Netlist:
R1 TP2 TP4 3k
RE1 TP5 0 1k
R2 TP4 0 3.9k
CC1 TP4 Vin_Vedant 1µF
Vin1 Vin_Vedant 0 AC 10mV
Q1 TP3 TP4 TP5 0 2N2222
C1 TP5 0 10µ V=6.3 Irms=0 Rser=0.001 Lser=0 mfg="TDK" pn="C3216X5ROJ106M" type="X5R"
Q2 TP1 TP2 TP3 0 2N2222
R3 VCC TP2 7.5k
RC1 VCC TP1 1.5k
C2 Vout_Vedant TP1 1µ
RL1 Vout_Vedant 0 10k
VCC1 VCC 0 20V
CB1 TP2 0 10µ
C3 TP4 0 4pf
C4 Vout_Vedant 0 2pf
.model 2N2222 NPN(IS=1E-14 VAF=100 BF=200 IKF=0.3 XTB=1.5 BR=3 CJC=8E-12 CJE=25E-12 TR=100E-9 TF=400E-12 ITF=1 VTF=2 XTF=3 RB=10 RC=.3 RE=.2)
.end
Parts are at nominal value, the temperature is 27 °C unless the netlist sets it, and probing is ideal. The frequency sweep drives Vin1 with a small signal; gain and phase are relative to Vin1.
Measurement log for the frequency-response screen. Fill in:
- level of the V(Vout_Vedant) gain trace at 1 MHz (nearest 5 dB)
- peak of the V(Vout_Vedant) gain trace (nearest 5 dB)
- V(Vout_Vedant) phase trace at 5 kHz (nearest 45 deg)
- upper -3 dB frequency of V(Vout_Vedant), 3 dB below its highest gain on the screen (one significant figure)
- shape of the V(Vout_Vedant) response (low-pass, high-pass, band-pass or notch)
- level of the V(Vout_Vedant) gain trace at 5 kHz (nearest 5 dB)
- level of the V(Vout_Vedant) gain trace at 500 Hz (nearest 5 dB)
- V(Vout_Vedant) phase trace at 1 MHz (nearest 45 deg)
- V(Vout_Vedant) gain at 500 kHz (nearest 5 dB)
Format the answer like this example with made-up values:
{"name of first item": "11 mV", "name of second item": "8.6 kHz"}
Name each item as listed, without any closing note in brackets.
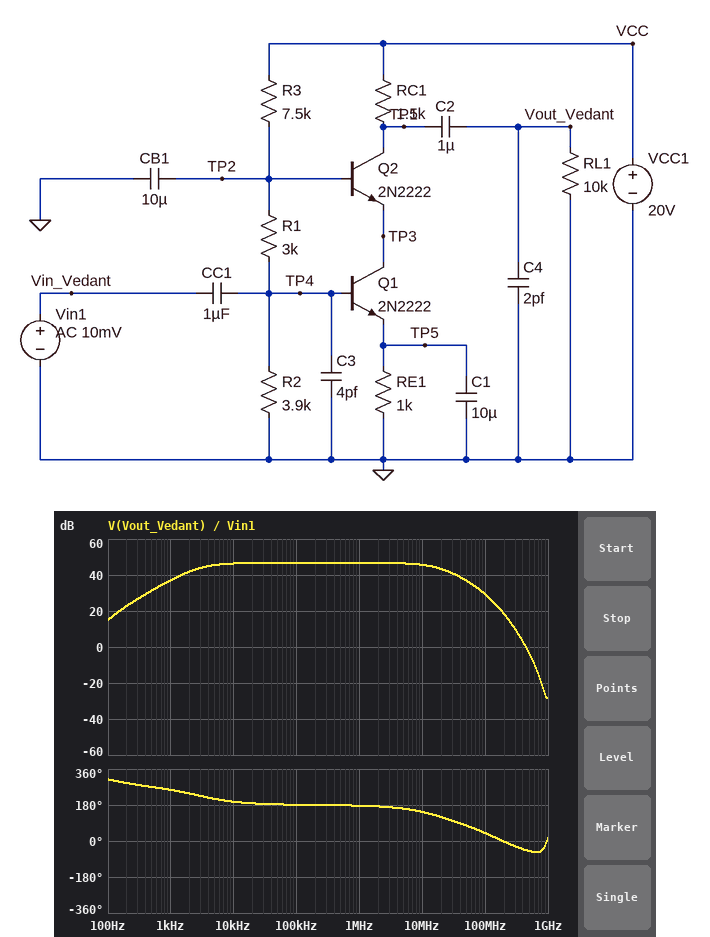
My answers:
{"level of the V(Vout_Vedant) gain trace at 1 MHz": "45 dB", "peak of the V(Vout_Vedant) gain trace": "45 dB", "V(Vout_Vedant) phase trace at 5 kHz": "225 deg", "upper -3 dB frequency of V(Vout_Vedant), 3 dB below its highest gain on the screen": "20 MHz", "shape of the V(Vout_Vedant) response": "band-pass", "level of the V(Vout_Vedant) gain trace at 5 kHz": "45 dB", "level of the V(Vout_Vedant) gain trace at 500 Hz": "30 dB", "V(Vout_Vedant) phase trace at 1 MHz": "180 deg", "V(Vout_Vedant) gain at 500 kHz": "45 dB"}
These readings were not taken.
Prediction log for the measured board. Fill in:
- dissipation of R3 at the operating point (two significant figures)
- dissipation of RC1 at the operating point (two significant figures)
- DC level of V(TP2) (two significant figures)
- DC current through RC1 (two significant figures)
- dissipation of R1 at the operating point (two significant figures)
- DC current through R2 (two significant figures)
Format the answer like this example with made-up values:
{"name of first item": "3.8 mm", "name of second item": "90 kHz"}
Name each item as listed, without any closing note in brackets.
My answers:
{"dissipation of R3 at the operating point": "15 mW", "dissipation of RC1 at the operating point": "31 mW", "DC level of V(TP2)": "9.5 V", "DC current through RC1": "4.6 mA", "dissipation of R1 at the operating point": "5.7 mW", "DC current through R2": "1.4 mA"}
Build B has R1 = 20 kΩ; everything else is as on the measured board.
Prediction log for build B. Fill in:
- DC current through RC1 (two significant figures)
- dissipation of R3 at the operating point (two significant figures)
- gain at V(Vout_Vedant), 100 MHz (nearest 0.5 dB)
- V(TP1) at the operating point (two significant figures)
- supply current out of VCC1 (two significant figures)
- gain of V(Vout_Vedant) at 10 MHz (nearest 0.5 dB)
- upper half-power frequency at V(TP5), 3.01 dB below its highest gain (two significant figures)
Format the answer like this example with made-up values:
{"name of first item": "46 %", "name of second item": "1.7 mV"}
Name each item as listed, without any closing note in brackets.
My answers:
{"DC current through RC1": "1.8 mA", "dissipation of R3 at the operating point": "3.1 mW", "gain at V(Vout_Vedant), 100 MHz": "21.0 dB", "V(TP1) at the operating point": "17 V", "supply current out of VCC1": "2.4 mA", "gain of V(Vout_Vedant) at 10 MHz": "37.5 dB", "upper half-power frequency at V(TP5), 3.01 dB below its highest gain": "1.2 kHz"}
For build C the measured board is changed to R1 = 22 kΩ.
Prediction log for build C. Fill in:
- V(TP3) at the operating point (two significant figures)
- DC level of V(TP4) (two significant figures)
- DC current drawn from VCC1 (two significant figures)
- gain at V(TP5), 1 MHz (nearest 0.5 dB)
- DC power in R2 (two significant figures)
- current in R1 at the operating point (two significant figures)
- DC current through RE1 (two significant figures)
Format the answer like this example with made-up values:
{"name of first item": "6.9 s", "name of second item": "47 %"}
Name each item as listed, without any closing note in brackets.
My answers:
{"V(TP3) at the operating point": "15 V", "DC level of V(TP4)": "2.3 V", "DC current drawn from VCC1": "2.2 mA", "gain at V(TP5), 1 MHz": "-60.0 dB", "DC power in R2": "1.4 mW", "current in R1 at the operating point": "600 µA", "DC current through RE1": "1.6 mA"}
